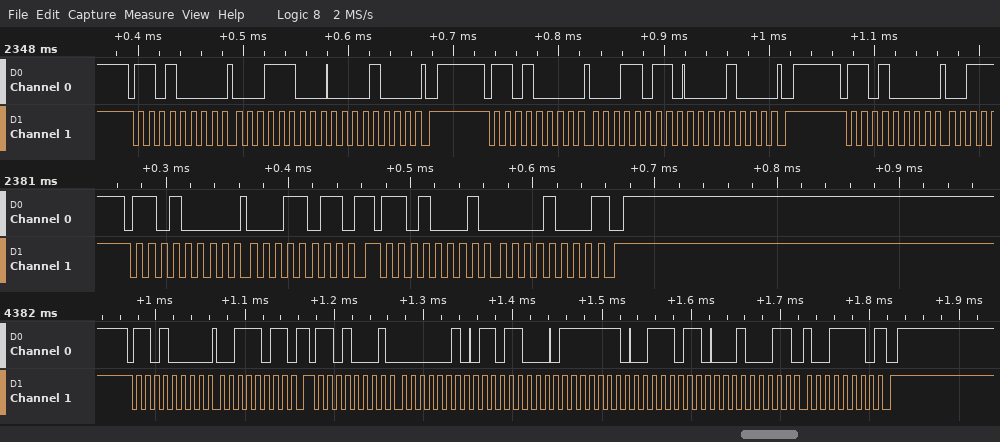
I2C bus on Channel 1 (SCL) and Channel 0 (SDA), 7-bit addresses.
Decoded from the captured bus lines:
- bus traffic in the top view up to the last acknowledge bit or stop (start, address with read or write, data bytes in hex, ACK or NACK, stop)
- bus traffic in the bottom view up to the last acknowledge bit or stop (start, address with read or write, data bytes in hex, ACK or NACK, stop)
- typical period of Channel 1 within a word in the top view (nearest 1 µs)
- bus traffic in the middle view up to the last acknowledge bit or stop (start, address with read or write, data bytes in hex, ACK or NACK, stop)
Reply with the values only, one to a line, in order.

start, address 68 write ACK, 1C ACK, 08 ACK, stop, start, address 68 write ACK, 1B ACK, 08 ACK, stop, start, address 68 write ACK
start, address 68 write ACK, 3B ACK, repeated start, address 68 read ACK, 02 ACK, D8 ACK, FE ACK, 76 ACK, 23 ACK, 9E NACK, stop
10 µs
start, address 68 write ACK, 1B ACK, repeated start, address 68 read ACK, 08 NACK, stop
